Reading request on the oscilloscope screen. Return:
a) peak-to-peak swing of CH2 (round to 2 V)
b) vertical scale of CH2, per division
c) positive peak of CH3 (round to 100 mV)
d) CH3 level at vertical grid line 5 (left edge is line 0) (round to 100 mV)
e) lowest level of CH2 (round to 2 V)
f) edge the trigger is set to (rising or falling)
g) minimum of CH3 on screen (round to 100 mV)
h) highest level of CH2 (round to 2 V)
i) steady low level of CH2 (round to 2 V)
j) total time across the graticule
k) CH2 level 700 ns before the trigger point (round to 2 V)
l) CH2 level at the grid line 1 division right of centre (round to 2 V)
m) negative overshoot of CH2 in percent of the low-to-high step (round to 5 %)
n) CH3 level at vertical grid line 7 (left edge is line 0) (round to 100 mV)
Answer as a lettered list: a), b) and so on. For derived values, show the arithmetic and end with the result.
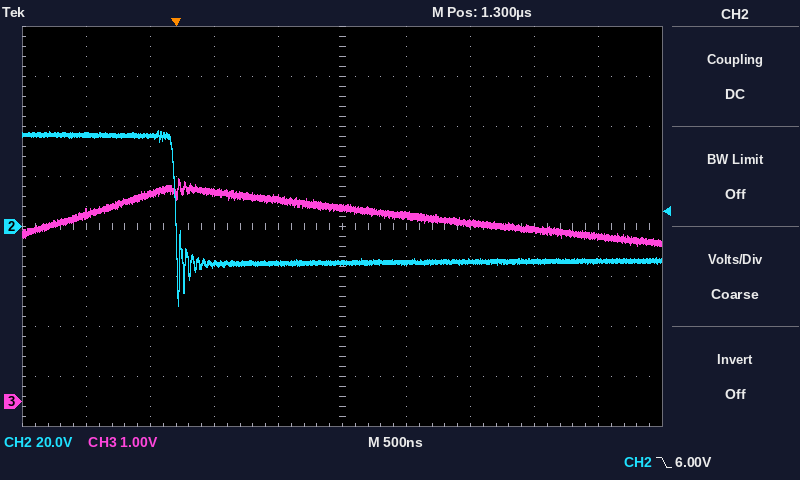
a) 38 V − (-32 V) = 70 V
b) 20 V
c) 4.5 V
d) 3.9 V
e) -32 V
f) falling
g) 3.1 V
h) 38 V
i) -14 V
j) 5 µs
k) 36 V
l) -14 V
m) 35 %
n) 3.6 V
